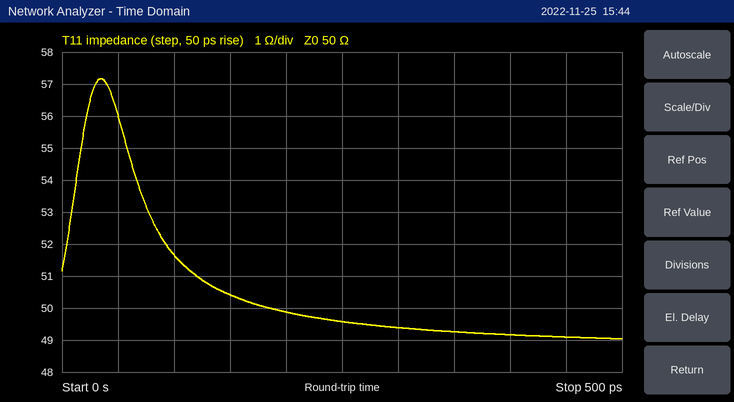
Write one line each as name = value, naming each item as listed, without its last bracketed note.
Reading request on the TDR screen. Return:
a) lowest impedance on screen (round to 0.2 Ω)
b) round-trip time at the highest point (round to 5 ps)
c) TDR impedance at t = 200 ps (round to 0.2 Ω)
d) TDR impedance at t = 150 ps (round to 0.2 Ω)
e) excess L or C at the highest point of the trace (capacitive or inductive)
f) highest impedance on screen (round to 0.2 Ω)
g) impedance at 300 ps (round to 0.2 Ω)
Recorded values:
lowest impedance on screen = 49.0 Ω
round-trip time at the highest point = 35 ps
TDR impedance at t = 200 ps = 49.8 Ω
TDR impedance at t = 150 ps = 50.4 Ω
excess L or C at the highest point of the trace = inductive
highest impedance on screen = 57.2 Ω
impedance at 300 ps = 49.4 Ω
